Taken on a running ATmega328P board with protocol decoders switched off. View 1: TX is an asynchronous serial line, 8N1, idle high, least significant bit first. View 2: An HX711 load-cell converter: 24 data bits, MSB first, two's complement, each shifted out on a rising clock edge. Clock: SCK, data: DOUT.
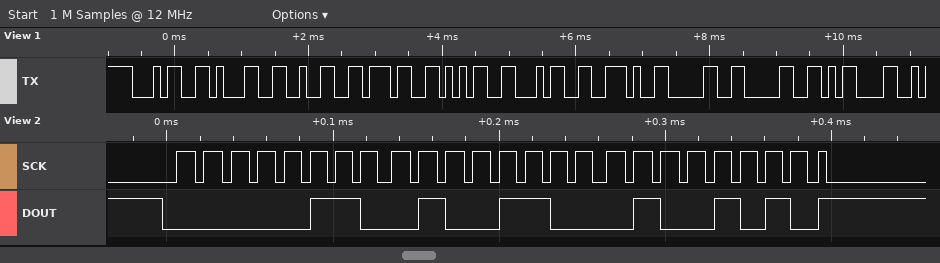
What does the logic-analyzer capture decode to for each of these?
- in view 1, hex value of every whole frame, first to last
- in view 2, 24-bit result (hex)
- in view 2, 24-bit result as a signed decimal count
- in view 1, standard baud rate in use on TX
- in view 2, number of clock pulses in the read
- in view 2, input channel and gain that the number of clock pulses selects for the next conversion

0x34 0x31 0x32 0x37 0x35 0x34 0x2E 0x30 0x30 0x0D
0x064C4A
412746
9600 baud
25
channel A, gain 128
